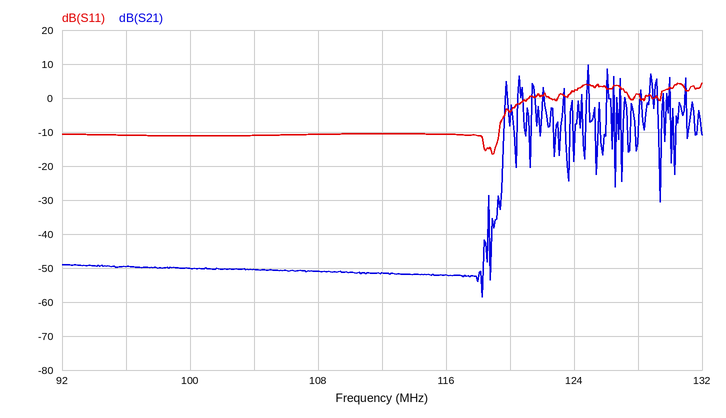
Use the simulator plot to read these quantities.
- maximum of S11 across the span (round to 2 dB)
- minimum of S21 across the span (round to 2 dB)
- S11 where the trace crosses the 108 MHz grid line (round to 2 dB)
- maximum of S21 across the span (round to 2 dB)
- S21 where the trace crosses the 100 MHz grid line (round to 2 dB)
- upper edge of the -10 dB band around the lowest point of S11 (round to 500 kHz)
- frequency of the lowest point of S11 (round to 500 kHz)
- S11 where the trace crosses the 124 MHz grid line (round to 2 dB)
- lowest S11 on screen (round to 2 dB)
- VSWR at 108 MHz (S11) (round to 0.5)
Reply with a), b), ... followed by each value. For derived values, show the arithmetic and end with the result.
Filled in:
a) 4 dB
b) -58 dB
c) -10 dB
d) 10 dB
e) -50 dB
f) 119.5 MHz
g) 119.0 MHz
h) 2 dB
i) -16 dB
j) |Γ| = 10^(-10/20) = 0.3162; VSWR = (1 + 0.3162)/(1 − 0.3162) ≈ 1.92, so 2.0 to the nearest 0.5
